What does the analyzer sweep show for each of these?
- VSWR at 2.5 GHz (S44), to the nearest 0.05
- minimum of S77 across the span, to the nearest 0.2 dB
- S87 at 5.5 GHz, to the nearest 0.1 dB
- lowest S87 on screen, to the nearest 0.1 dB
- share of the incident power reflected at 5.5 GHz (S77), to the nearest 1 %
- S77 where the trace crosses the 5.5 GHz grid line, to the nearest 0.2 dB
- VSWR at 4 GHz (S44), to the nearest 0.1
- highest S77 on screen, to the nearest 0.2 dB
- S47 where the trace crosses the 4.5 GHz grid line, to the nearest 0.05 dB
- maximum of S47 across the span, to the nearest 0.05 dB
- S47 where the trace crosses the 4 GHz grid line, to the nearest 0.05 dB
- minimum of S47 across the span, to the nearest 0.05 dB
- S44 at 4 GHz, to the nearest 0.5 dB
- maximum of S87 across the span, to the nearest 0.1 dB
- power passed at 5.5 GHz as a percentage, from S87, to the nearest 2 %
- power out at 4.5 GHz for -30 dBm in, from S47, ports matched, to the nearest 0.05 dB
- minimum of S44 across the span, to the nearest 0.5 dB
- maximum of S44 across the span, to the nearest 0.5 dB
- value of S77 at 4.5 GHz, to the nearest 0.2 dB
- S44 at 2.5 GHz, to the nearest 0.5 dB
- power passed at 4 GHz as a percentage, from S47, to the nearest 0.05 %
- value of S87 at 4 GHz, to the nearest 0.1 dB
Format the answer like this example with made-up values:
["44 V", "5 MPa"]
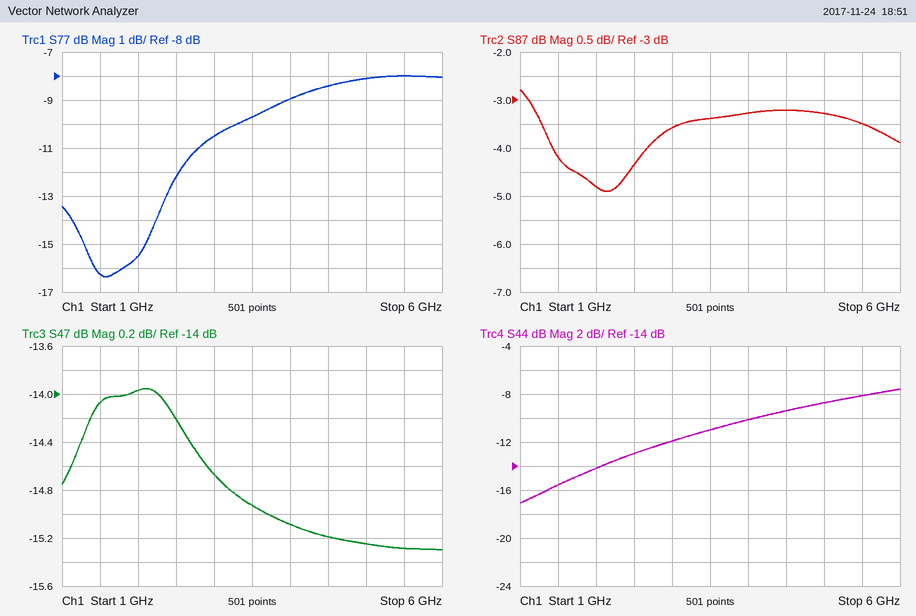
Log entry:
["1.60", "-16.4 dB", "-3.5 dB", "-4.9 dB", "16 %", "-8.0 dB", "1.9", "-8.0 dB", "-15.20 dB", "-13.95 dB", "-15.10 dB", "-15.30 dB", "-10.0 dB", "-2.8 dB", "44 %", "-45.20 dBm", "-17.0 dB", "-7.5 dB", "-8.4 dB", "-13.0 dB", "3.10 %", "-3.3 dB"]
